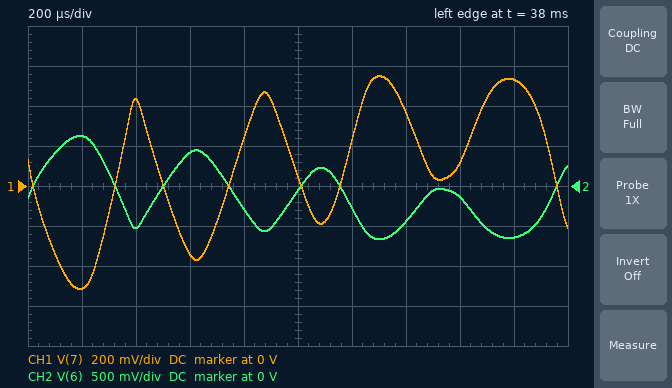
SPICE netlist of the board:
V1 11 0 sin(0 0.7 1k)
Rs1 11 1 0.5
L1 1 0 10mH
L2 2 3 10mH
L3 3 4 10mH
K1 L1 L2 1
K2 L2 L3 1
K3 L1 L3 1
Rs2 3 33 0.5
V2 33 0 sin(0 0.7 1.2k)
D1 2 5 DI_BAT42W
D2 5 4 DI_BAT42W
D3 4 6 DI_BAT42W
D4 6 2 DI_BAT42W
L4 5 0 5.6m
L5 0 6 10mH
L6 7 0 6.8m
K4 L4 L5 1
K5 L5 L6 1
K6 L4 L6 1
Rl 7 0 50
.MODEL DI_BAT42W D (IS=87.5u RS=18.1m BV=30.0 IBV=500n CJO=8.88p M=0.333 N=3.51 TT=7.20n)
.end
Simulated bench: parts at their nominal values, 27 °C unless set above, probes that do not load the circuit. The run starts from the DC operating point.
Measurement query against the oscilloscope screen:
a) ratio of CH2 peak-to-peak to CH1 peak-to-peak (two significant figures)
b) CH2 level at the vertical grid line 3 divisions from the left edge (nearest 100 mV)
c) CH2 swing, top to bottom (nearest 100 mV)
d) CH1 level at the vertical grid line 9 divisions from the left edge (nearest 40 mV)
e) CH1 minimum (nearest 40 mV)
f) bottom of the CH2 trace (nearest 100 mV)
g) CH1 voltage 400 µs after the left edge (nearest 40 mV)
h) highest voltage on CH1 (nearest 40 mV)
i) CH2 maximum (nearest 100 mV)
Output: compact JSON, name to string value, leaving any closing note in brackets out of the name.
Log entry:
{"ratio of CH2 peak-to-peak to CH1 peak-to-peak": "1.2", "CH2 level at the vertical grid line 3 divisions from the left edge": "400 mV", "CH2 swing, top to bottom": "1.3 V", "CH1 level at the vertical grid line 9 divisions from the left edge": "520 mV", "CH1 minimum": "-520 mV", "bottom of the CH2 trace": "-700 mV", "CH1 voltage 400 µs after the left edge": "440 mV", "highest voltage on CH1": "560 mV", "CH2 maximum": "600 mV"}
